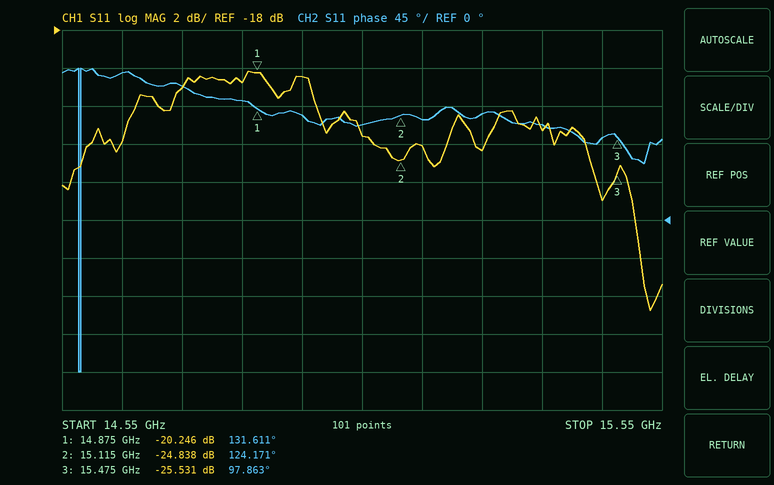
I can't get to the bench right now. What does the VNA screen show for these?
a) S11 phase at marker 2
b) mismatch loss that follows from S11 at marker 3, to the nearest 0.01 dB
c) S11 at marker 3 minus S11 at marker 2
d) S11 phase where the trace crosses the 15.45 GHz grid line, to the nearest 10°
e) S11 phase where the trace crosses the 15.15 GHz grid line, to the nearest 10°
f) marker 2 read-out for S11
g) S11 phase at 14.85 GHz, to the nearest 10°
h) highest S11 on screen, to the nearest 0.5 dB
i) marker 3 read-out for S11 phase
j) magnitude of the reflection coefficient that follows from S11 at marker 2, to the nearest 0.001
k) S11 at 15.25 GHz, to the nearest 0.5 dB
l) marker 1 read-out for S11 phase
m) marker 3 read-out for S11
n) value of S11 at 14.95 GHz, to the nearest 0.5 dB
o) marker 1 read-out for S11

124.171°
0.01 dB
-0.693 dB
100°
120°
-24.838 dB
140°
-20.0 dB
97.863°
0.057
-24.5 dB
131.611°
-25.531 dB
-20.5 dB
-20.246 dB
